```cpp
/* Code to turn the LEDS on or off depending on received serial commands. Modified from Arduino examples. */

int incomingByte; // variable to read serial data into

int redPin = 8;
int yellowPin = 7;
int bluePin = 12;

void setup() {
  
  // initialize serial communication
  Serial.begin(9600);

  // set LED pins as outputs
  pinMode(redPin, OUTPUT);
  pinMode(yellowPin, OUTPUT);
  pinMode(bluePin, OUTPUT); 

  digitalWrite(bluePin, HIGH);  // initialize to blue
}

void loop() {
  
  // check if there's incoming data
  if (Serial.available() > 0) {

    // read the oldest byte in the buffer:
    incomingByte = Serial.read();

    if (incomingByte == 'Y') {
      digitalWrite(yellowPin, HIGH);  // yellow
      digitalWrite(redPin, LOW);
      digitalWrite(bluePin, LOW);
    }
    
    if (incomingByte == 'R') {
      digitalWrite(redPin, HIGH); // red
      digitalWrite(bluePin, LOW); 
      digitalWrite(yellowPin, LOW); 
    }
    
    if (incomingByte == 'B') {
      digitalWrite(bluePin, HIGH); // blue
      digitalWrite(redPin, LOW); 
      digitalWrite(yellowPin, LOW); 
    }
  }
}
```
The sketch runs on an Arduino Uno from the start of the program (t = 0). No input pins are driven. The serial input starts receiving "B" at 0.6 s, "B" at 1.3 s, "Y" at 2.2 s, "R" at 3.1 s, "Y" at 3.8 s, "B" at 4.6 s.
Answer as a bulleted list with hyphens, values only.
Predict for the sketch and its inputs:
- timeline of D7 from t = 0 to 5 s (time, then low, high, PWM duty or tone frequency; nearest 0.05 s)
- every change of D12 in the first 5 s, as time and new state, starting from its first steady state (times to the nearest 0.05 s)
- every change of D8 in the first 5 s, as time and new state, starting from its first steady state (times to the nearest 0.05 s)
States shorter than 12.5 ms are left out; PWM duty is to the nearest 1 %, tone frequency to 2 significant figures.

- 0 s low; 2.2 s high; 3.1 s low; 3.8 s high; 4.6 s low
- 0 s high; 2.2 s low; 4.6 s high
- 0 s low; 3.1 s high; 3.8 s low
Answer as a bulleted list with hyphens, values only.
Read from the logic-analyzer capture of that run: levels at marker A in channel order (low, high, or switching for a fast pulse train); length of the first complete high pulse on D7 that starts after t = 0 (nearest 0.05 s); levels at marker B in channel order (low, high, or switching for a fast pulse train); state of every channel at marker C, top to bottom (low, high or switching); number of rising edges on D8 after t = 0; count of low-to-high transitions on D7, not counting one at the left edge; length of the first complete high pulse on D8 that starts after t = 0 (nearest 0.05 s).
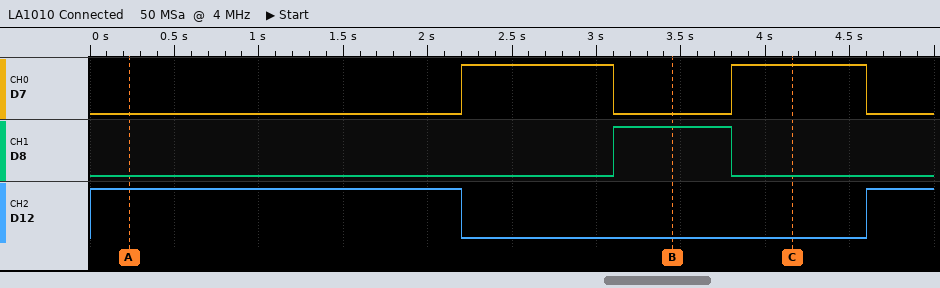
- D7 low, D8 low, D12 high
- 0.90 s
- D7 low, D8 high, D12 low
- D7 high, D8 low, D12 low
- 1
- 2
- 0.70 s
